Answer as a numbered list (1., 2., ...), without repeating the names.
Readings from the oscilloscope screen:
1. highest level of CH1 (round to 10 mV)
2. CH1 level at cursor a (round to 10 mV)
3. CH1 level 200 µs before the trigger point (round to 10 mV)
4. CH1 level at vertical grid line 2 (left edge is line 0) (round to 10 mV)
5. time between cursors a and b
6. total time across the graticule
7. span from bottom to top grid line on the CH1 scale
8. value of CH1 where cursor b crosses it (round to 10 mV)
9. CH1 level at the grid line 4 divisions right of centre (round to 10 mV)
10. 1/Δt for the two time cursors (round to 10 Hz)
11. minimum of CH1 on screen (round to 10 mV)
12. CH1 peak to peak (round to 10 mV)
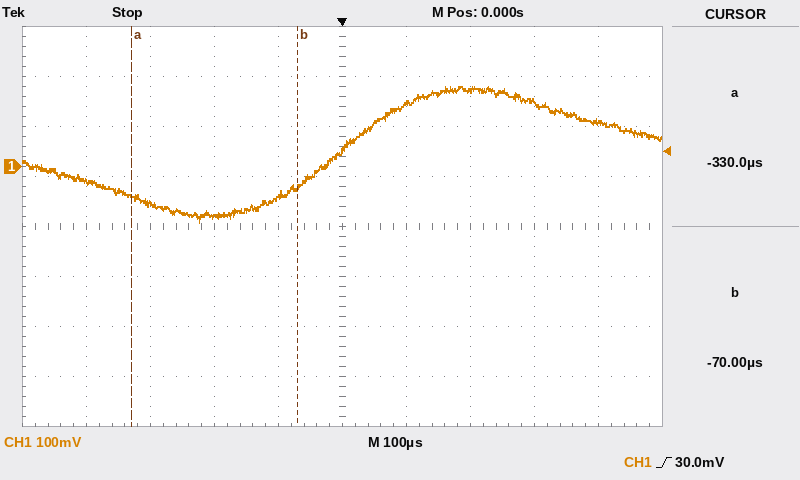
1. 160 mV
2. -60 mV
3. -100 mV
4. -70 mV
5. 260 µs
6. 1 ms
7. 800 mV
8. -40 mV
9. 90 mV
10. 3.85 kHz
11. -110 mV
12. 270 mV
